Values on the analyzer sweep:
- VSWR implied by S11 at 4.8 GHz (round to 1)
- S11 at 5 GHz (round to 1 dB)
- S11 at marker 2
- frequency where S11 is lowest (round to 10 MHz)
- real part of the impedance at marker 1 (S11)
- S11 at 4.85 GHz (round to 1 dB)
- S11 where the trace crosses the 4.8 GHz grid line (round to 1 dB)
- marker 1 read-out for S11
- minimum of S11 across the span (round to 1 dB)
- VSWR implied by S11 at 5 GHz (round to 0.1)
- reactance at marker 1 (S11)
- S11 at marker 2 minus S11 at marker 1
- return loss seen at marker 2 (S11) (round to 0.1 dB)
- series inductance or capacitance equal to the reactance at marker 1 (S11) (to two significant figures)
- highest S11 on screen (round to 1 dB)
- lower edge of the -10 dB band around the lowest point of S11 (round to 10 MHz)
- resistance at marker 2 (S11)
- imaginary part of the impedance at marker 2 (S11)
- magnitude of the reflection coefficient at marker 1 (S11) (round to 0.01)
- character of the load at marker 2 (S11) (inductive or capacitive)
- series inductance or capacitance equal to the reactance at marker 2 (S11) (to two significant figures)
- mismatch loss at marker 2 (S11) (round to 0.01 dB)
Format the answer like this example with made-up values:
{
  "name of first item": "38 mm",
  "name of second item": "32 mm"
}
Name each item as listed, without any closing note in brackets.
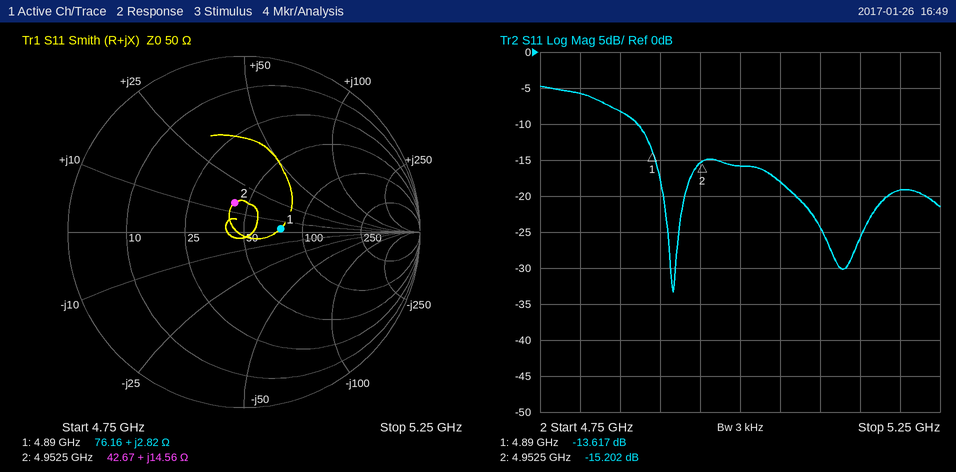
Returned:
{
  "VSWR implied by S11 at 4.8 GHz": "3",
  "S11 at 5 GHz": "-16 dB",
  "S11 at marker 2": "-15.202 dB",
  "frequency where S11 is lowest": "4.92 GHz",
  "real part of the impedance at marker 1": "76.16 Ω",
  "S11 at 4.85 GHz": "-8 dB",
  "S11 where the trace crosses the 4.8 GHz grid line": "-6 dB",
  "marker 1 read-out for S11": "-13.617 dB",
  "minimum of S11 across the span": "-33 dB",
  "VSWR implied by S11 at 5 GHz": "1.4",
  "reactance at marker 1": "+2.82 Ω",
  "S11 at marker 2 minus S11 at marker 1": "-1.585 dB",
  "return loss seen at marker 2 (S11)": "15.2 dB",
  "series inductance or capacitance equal to the reactance at marker 1 (S11)": "92 pH",
  "highest S11 on screen": "-5 dB",
  "lower edge of the -10 dB band around the lowest point of S11": "4.87 GHz",
  "resistance at marker 2": "42.67 Ω",
  "imaginary part of the impedance at marker 2": "+14.56 Ω",
  "magnitude of the reflection coefficient at marker 1 (S11)": "0.21",
  "character of the load at marker 2 (S11)": "inductive",
  "series inductance or capacitance equal to the reactance at marker 2 (S11)": "470 pH",
  "mismatch loss at marker 2 (S11)": "0.13 dB"
}
